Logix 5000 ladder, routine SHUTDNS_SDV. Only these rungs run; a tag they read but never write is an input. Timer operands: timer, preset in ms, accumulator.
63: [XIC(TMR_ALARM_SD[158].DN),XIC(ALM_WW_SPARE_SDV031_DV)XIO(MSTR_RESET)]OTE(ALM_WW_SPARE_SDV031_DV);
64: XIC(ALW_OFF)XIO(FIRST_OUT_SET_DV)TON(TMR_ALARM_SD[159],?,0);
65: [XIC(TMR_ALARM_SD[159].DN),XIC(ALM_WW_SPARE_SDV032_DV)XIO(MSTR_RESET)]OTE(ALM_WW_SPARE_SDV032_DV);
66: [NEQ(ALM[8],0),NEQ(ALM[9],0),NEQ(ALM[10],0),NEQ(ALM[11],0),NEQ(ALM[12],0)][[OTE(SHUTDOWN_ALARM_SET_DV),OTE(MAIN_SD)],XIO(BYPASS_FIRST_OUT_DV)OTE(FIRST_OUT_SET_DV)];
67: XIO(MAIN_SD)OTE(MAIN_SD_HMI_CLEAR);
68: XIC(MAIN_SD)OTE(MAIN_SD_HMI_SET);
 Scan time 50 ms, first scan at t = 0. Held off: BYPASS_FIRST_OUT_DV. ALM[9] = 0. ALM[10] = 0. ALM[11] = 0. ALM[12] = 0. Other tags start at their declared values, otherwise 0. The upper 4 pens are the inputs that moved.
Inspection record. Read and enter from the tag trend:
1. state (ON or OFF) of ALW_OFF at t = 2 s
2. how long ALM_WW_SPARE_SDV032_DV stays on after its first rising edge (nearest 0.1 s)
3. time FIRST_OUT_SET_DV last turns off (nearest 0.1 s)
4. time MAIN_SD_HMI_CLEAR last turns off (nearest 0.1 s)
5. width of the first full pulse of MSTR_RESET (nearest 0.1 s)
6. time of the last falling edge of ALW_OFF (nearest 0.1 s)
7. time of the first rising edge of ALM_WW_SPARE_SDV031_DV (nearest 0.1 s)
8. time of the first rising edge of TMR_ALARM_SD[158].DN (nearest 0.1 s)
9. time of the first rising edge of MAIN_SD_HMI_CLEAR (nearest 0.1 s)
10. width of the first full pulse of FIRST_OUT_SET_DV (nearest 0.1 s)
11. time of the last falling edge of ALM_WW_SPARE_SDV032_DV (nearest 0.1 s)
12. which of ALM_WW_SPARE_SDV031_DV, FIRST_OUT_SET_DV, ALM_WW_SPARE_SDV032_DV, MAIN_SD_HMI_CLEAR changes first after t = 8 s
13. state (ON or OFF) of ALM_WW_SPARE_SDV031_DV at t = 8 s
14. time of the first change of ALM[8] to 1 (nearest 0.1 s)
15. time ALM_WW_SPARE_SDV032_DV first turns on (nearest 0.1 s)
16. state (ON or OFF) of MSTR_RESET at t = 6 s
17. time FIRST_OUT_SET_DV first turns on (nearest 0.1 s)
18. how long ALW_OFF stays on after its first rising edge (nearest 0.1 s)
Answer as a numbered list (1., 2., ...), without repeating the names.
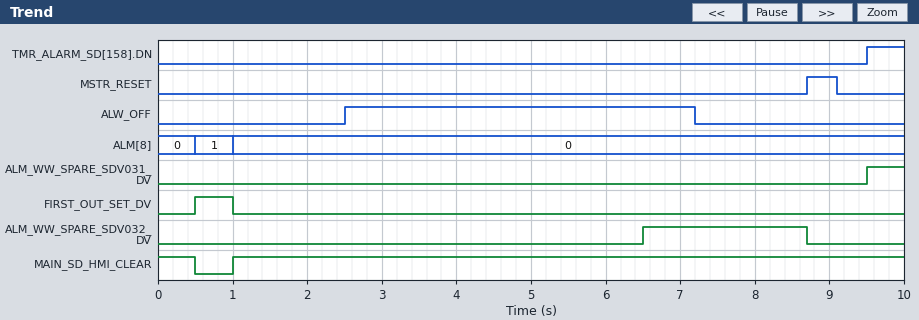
1. OFF
2. 2.2 s
3. 1.0 s
4. 0.5 s
5. 0.4 s
6. 7.2 s
7. 9.5 s
8. 9.5 s
9. 1.0 s
10. 0.5 s
11. 8.7 s
12. ALM_WW_SPARE_SDV032_DV
13. OFF
14. 0.5 s
15. 6.5 s
16. OFF
17. 0.5 s
18. 4.7 s
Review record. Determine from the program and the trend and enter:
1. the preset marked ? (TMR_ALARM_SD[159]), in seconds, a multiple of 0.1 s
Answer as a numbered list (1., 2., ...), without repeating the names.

1. 4.0 s
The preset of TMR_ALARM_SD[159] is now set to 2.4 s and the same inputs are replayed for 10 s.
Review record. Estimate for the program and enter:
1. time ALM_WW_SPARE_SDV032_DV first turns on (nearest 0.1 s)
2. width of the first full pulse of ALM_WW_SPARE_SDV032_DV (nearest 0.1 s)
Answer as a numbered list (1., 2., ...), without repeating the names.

1. 4.9 s
2. 3.8 s
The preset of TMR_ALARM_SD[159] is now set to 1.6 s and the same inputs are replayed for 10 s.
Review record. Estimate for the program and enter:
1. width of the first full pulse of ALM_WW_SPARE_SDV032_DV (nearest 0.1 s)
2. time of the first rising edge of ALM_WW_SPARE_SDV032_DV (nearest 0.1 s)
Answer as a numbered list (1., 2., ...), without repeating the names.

1. 4.6 s
2. 4.1 s
